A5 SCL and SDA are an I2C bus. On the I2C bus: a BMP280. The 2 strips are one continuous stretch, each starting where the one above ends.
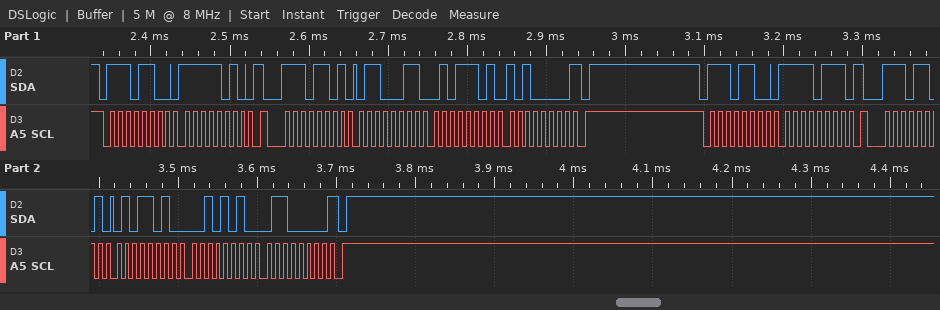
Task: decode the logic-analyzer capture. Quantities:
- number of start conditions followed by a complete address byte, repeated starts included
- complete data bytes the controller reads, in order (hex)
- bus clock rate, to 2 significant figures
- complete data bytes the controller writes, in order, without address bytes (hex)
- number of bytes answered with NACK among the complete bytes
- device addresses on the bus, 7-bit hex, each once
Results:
4
63 5D A0 5A 2A 60
100 kHz
FA F7
2
0x76
